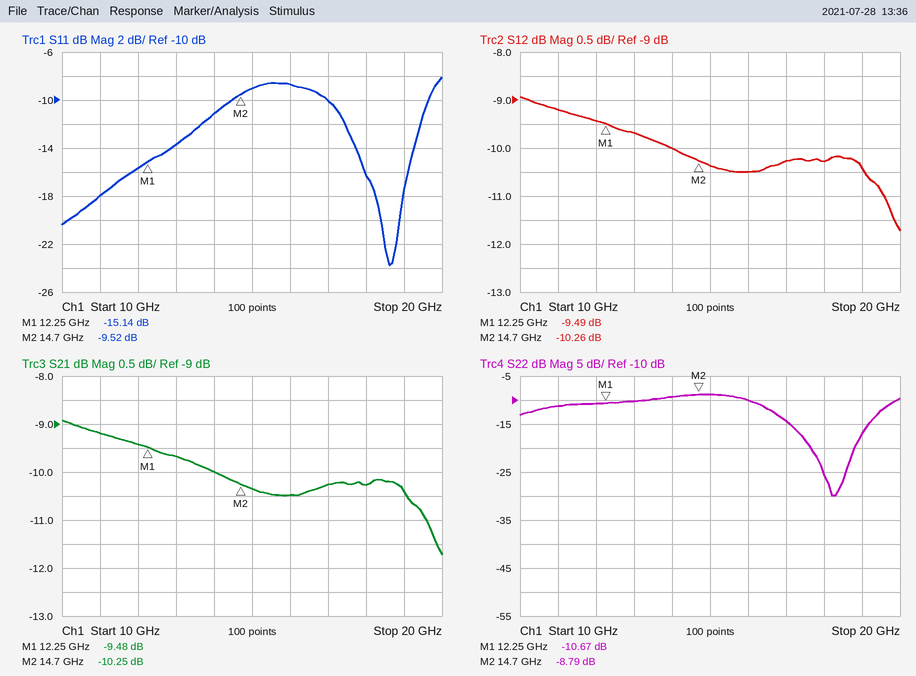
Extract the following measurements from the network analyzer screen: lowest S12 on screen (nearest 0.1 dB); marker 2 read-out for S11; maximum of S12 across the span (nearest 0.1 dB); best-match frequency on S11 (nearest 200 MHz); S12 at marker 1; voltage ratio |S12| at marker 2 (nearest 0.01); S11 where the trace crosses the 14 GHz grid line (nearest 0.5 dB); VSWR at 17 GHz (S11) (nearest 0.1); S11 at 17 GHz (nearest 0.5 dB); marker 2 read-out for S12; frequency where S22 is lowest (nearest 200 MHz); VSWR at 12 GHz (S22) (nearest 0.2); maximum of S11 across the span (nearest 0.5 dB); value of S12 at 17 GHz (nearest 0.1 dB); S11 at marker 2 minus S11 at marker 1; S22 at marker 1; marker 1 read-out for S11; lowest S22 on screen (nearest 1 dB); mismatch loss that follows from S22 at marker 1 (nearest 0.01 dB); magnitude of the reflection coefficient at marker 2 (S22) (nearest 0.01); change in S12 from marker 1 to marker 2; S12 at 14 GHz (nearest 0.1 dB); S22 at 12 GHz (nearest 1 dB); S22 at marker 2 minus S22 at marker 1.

-11.7 dB
-9.52 dB
-8.9 dB
18.6 GHz
-9.49 dB
0.31
-11.0 dB
1.9
-10.0 dB
-10.26 dB
18.2 GHz
1.8
-8.0 dB
-10.3 dB
5.62 dB
-10.67 dB
-15.14 dB
-30 dB
0.39 dB
0.36
-0.77 dB
-10.0 dB
-11 dB
1.88 dB
